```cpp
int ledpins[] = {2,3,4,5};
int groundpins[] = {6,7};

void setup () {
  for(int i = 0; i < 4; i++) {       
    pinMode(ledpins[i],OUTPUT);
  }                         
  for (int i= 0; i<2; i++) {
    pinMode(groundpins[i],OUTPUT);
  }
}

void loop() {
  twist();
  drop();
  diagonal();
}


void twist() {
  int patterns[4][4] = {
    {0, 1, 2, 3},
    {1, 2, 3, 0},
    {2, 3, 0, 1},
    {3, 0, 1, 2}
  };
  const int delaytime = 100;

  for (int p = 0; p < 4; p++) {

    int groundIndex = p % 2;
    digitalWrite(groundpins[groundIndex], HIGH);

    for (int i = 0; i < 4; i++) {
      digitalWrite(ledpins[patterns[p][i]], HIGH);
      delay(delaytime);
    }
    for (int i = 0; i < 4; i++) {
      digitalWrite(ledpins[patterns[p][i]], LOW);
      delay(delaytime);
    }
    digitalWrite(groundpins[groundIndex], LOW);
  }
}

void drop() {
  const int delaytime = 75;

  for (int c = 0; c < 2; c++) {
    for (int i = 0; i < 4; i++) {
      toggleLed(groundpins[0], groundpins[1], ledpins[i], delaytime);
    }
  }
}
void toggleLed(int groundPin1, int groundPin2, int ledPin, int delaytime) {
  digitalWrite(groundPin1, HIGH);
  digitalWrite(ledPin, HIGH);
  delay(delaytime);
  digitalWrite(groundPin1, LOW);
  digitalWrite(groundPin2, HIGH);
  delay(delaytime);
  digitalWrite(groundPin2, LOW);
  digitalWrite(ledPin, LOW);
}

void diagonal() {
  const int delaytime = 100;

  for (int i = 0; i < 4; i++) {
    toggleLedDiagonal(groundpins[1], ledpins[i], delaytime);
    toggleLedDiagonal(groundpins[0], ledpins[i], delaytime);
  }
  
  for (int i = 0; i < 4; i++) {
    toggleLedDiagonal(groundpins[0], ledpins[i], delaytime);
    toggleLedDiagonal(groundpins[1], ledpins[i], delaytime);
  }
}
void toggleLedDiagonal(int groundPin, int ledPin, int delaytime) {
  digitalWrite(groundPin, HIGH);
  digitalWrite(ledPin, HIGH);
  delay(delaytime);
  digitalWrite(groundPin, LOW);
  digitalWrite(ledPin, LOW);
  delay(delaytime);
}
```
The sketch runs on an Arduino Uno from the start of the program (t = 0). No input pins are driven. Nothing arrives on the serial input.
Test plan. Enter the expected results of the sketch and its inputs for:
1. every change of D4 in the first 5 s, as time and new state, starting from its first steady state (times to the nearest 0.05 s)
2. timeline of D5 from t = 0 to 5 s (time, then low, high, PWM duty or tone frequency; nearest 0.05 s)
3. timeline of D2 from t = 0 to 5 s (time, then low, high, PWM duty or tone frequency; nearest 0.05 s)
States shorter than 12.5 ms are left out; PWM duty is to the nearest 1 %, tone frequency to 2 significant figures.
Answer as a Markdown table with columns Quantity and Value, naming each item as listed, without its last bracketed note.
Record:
| Quantity | Value |
|---|---|
| every change of D4 in the first 5 s, as time and new state, starting from its first steady state | 0 s low; 0.2 s high; 0.6 s low; 0.9 s high; 1.3 s low; 1.6 s high; 2 s low; 2.7 s high; 3.1 s low; 3.5 s high; 3.65 s low; 4.1 s high; 4.25 s low |
| timeline of D5 from t = 0 to 5 s | 0 s low; 0.3 s high; 0.7 s low; 1 s high; 1.4 s low; 1.7 s high; 2.1 s low; 2.4 s high; 2.8 s low; 3.65 s high; 3.8 s low; 4.25 s high; 4.4 s low |
| timeline of D2 from t = 0 to 5 s | 0 s high; 0.4 s low; 1.1 s high; 1.5 s low; 1.8 s high; 2.2 s low; 2.5 s high; 2.9 s low; 3.2 s high; 3.35 s low; 3.8 s high; 3.95 s low; 4.4 s high; 4.5 s low; 4.6 s high; 4.7 s low |
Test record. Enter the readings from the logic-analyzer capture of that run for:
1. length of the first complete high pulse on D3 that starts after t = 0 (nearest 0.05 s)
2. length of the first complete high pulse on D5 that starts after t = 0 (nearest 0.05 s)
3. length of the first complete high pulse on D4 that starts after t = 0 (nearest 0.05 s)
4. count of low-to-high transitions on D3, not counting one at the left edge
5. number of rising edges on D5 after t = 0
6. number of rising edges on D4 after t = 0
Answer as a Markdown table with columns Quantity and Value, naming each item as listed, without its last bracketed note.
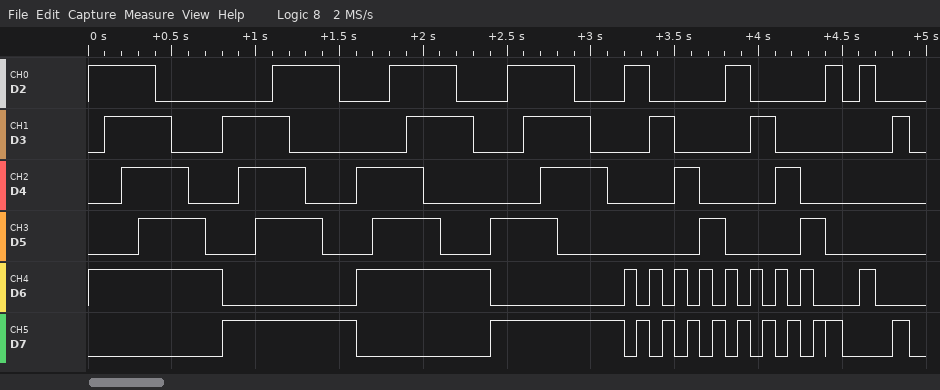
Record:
| Quantity | Value |
|---|---|
| length of the first complete high pulse on D3 that starts after t = 0 | 0.40 s |
| length of the first complete high pulse on D5 that starts after t = 0 | 0.40 s |
| length of the first complete high pulse on D4 that starts after t = 0 | 0.40 s |
| count of low-to-high transitions on D3, not counting one at the left edge | 7 |
| number of rising edges on D5 after t = 0 | 6 |
| number of rising edges on D4 after t = 0 | 6 |
